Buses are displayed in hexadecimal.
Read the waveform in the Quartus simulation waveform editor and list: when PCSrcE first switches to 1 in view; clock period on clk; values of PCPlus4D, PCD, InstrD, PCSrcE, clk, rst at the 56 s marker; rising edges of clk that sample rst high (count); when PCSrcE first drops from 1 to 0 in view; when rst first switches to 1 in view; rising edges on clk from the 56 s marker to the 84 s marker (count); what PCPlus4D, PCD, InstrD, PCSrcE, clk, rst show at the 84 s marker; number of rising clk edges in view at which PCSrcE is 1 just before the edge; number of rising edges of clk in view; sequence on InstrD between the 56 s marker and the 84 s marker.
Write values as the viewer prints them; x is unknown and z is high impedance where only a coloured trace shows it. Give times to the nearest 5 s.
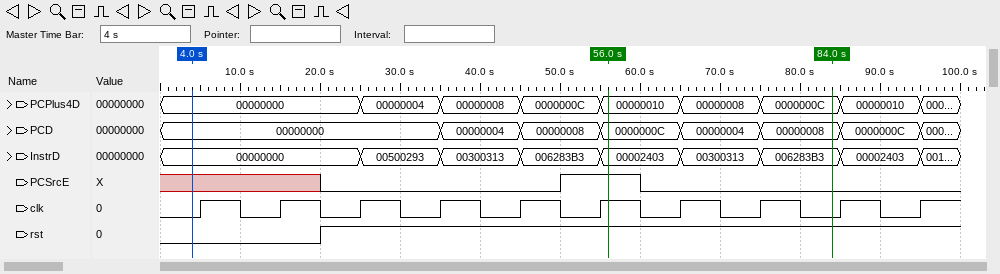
50 s
10 s
PCPlus4D=00000010, PCD=0000000C, InstrD=00002403, PCSrcE=1, clk=1, rst=1
8
60 s
20 s
2
PCPlus4D=0000000C, PCD=00000008, InstrD=006283B3, PCSrcE=0, clk=0, rst=1
1
10
00002403, 00300313, 006283B3
